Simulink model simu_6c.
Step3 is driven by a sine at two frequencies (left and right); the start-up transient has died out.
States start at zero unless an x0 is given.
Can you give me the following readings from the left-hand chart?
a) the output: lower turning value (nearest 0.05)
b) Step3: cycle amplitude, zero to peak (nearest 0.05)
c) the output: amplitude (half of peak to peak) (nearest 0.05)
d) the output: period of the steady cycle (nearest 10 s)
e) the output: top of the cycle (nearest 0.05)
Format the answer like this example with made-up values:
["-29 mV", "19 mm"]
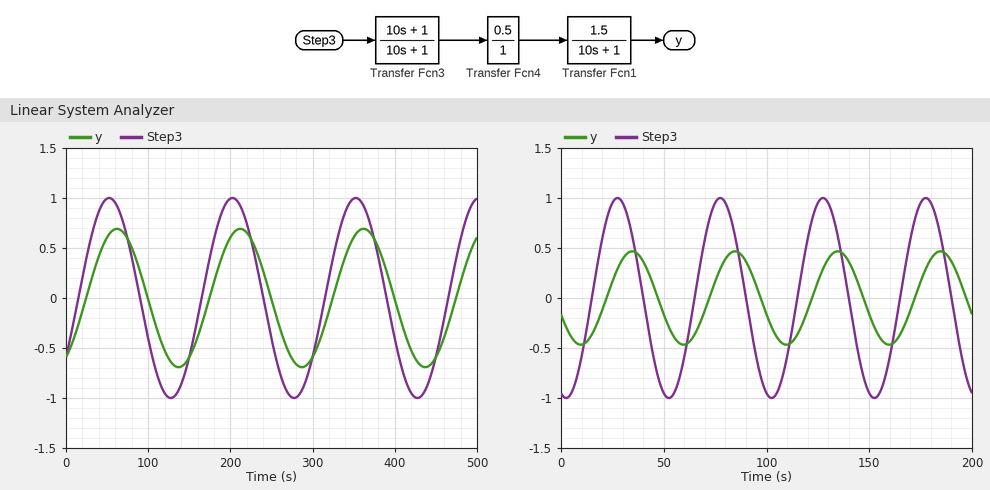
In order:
["-0.70", "1.00", "0.70", "150 s", "0.70"]
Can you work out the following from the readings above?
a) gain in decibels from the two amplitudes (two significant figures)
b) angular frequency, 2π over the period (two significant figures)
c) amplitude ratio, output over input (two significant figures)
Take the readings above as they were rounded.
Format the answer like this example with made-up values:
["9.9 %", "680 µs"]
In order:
["-3.1 dB", "0.042 rad/s", "0.70"]
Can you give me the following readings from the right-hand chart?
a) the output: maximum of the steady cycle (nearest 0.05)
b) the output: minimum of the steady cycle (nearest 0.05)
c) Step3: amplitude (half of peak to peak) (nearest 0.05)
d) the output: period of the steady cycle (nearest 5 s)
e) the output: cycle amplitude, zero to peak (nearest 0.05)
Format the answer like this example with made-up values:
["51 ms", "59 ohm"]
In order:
["0.45", "-0.45", "1.00", "50 s", "0.45"]
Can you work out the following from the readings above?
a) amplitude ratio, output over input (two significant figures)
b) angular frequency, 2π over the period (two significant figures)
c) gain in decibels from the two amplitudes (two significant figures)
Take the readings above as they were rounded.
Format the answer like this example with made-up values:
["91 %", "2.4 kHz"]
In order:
["0.45", "0.13 rad/s", "-6.9 dB"]
